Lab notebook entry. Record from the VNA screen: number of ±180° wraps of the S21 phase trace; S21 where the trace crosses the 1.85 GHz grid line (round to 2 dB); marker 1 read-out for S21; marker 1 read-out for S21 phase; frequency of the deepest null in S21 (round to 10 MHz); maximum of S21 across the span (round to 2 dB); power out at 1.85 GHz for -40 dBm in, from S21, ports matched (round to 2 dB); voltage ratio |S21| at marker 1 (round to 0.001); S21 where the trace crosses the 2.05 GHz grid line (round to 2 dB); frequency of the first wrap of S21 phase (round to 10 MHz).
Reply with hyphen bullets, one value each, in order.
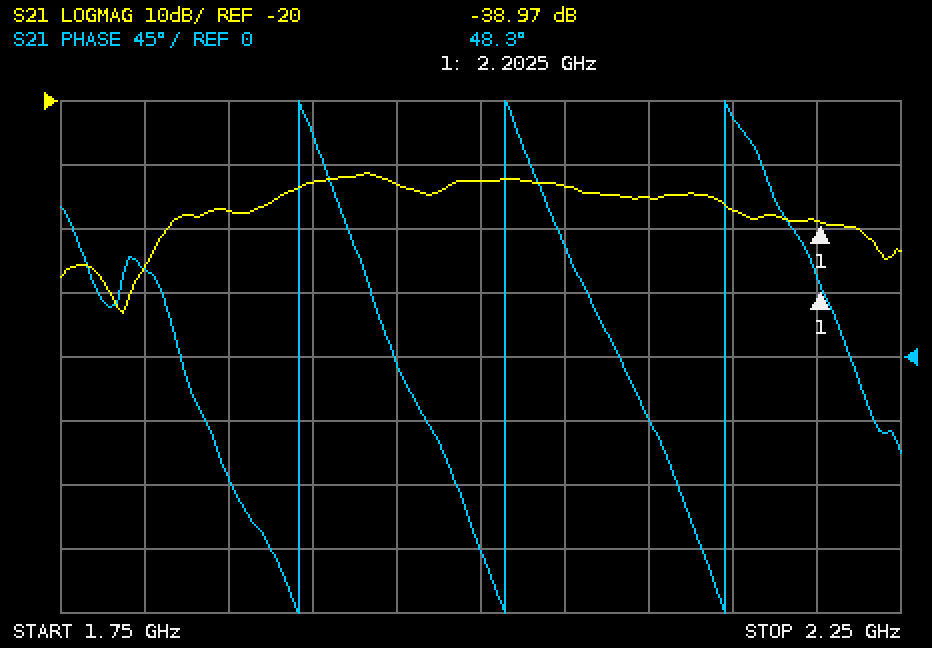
- 3
- -38 dB
- -38.97 dB
- 48.3°
- 1.79 GHz
- -32 dB
- -78 dBm
- 0.011
- -34 dB
- 1.89 GHz
